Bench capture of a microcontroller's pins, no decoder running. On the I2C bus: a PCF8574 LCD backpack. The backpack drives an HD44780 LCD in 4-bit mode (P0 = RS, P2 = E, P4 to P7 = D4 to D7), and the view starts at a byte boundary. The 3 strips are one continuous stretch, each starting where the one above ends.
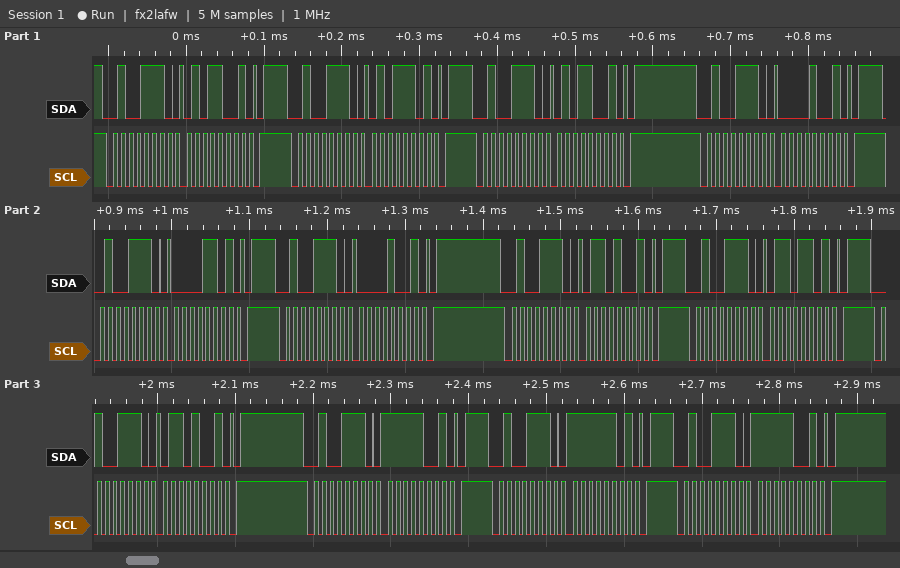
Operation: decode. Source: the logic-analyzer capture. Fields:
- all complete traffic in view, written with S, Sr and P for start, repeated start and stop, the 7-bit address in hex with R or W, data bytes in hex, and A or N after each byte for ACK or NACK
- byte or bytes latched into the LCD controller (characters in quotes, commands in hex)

S 27W A 59 A P S 27W A 5D A P S 27W A 59 A P S 27W A 09 A P S 27W A 0D A P S 27W A 09 A P S 27W A 69 A P S 27W A 6D A P S 27W A 69 A P S 27W A F9 A P S 27W A FD A P S 27W A F9 A P
'P' 'o'
